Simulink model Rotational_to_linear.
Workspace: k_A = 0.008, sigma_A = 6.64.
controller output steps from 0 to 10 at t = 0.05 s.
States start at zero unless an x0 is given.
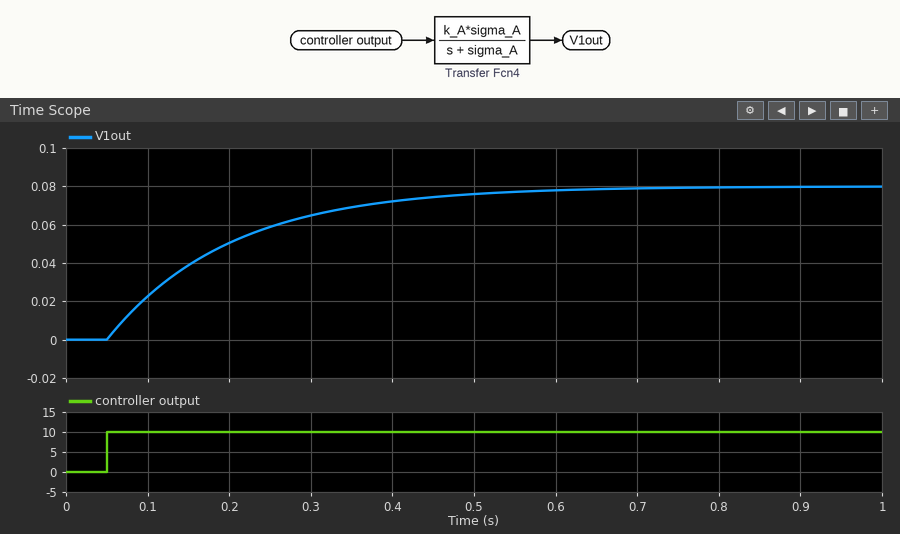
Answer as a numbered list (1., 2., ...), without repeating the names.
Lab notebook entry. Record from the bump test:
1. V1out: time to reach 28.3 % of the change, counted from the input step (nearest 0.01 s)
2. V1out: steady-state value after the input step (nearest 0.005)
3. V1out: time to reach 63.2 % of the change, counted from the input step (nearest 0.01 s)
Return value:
1. 0.05 s
2. 0.080
3. 0.15 s
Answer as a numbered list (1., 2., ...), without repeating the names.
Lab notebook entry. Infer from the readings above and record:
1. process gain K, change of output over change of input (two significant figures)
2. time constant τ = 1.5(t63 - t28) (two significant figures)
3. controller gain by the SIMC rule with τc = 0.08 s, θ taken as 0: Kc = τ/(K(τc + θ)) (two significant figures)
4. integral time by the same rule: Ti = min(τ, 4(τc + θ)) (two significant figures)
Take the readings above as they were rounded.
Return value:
1. 0.0080
2. 0.15 s
3. 230
4. 0.15 s
